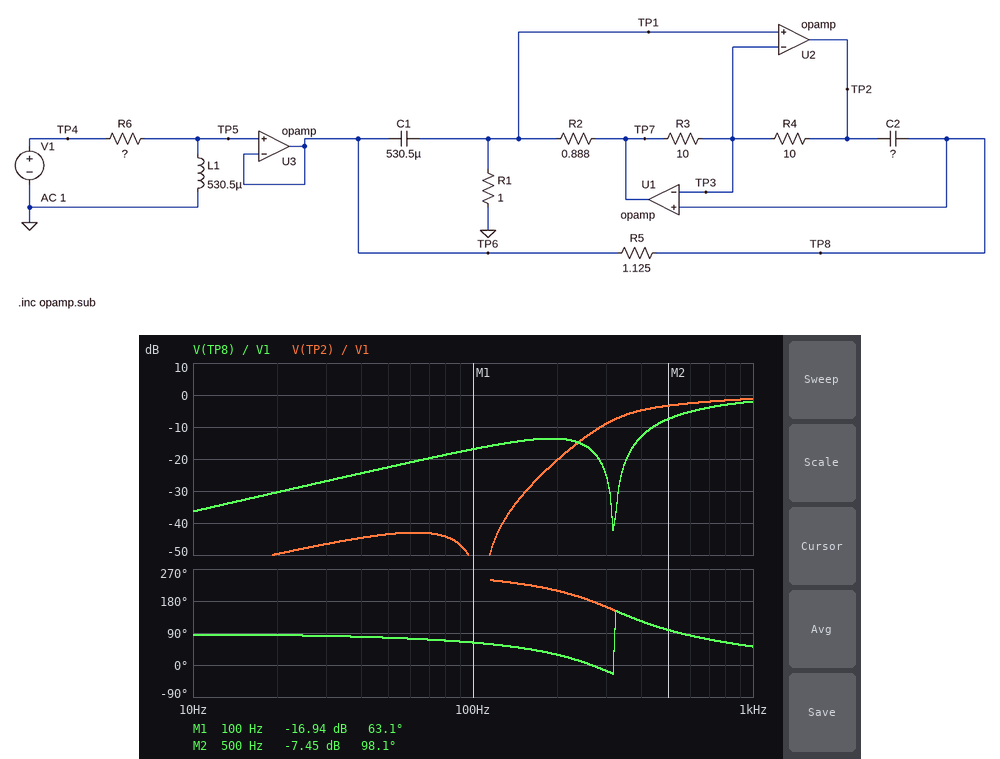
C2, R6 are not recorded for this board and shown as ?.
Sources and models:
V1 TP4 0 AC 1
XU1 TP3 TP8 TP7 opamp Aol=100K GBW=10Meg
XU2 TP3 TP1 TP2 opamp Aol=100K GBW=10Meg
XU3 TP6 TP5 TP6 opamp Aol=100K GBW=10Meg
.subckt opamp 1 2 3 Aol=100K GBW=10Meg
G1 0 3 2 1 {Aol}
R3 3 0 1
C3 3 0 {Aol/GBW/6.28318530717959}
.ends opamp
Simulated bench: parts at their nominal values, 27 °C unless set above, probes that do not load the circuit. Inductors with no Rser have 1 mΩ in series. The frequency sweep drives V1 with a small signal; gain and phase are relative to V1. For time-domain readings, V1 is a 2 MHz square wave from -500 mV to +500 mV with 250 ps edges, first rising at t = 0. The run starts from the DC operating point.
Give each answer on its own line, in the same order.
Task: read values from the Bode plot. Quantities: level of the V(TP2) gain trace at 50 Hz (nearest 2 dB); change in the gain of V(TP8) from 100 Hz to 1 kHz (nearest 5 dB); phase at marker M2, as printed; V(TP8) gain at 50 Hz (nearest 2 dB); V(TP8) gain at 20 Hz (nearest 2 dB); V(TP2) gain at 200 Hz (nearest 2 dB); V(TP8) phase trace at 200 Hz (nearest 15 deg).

-44 dB
15 dB
98.1 deg
-22 dB
-30 dB
-20 dB
30 deg
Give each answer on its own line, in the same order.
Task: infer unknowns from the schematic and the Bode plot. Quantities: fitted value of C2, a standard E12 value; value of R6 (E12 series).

470 µF
2.2 Ω
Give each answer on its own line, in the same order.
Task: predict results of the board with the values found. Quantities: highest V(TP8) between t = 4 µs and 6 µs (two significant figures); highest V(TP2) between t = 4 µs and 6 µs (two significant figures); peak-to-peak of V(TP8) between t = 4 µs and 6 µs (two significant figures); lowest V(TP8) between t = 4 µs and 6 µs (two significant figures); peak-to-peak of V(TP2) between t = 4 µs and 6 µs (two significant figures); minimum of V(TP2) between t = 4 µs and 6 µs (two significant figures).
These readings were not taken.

1.1 V
1.1 V
1.3 V
-160 mV
1.3 V
-160 mV
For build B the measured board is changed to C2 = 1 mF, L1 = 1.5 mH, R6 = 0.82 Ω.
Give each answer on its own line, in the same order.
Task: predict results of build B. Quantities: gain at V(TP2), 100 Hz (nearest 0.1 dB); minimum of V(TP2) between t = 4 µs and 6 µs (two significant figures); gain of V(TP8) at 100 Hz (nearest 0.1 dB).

-22.8 dB
-150 mV
-4.6 dB
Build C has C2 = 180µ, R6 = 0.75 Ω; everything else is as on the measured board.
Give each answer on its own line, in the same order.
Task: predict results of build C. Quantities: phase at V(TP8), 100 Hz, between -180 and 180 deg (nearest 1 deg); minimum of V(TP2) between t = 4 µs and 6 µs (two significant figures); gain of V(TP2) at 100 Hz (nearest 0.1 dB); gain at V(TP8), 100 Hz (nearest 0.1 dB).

59 deg
-150 mV
-30.1 dB
-7.9 dB
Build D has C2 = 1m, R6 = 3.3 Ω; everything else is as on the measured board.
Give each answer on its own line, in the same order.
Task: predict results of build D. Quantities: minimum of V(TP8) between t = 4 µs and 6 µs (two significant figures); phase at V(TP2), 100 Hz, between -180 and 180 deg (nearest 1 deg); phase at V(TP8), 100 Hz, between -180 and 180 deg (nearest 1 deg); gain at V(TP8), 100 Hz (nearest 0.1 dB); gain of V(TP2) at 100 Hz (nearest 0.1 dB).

-170 mV
-134 deg
46 deg
-22.1 dB
-40.3 dB
